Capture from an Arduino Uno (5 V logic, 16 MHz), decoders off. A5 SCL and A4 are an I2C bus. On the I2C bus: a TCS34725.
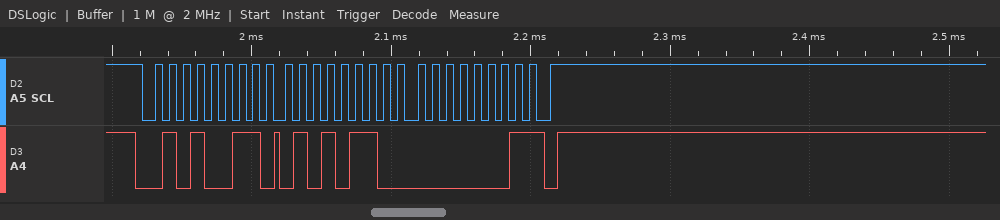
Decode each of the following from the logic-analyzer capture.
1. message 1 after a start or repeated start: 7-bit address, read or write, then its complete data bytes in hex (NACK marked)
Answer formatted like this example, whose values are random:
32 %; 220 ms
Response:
0x29 read: 56 01 NACK
